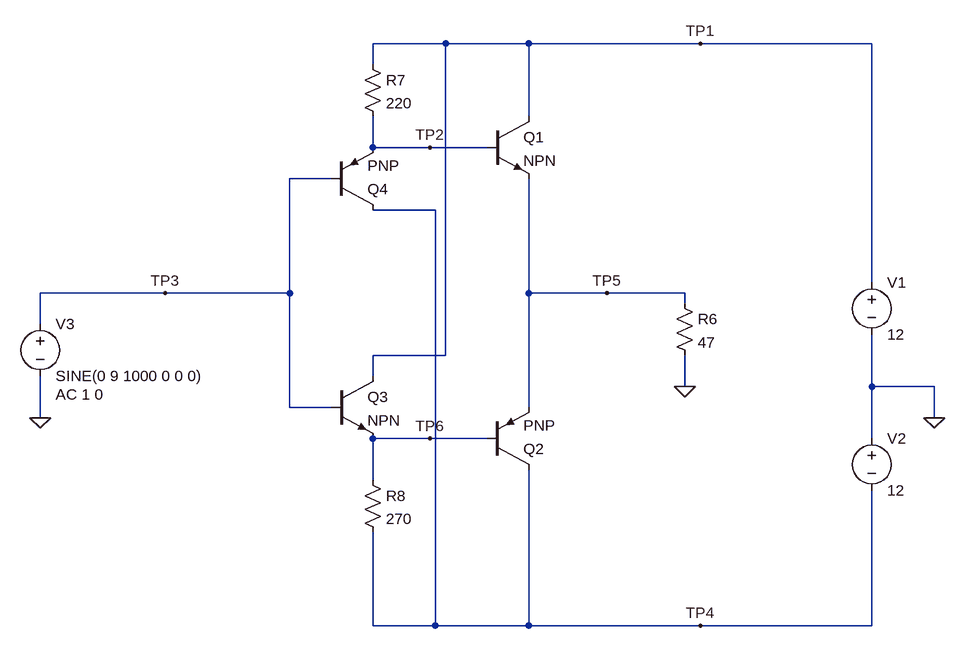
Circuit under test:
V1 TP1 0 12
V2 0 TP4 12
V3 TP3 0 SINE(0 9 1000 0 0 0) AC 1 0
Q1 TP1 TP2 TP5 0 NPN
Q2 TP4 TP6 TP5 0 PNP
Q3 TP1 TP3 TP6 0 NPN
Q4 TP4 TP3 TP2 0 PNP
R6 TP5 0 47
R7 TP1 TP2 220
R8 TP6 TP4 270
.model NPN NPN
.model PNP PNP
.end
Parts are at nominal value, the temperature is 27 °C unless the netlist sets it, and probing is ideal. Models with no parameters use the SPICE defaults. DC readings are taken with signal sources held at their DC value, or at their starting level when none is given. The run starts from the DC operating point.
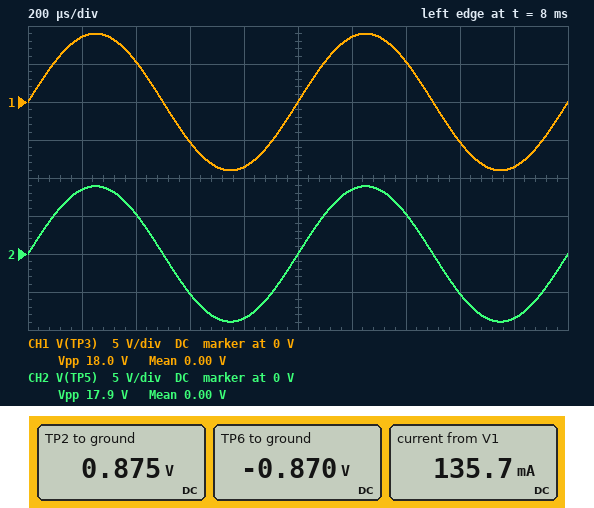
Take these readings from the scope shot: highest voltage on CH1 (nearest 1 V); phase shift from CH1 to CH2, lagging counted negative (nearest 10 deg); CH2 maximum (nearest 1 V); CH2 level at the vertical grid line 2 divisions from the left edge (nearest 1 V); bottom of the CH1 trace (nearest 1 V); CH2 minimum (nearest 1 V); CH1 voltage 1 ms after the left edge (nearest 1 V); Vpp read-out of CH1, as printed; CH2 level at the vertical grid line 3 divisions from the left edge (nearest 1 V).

9 V
0 deg
9 V
5 V
-9 V
-9 V
0 V
18.0 V
-5 V
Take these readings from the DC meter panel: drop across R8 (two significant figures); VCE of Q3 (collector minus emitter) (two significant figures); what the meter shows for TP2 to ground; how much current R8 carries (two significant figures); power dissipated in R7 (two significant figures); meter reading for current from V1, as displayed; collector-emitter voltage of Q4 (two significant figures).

11 V
13 V
0.875 V
41 mA
560 mW
135.7 mA
-13 V
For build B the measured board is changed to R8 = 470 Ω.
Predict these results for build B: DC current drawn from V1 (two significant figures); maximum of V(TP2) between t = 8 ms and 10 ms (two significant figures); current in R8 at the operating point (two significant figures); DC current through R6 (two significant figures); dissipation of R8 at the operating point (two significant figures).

110 mA
9.8 V
24 mA
210 µA
260 mW
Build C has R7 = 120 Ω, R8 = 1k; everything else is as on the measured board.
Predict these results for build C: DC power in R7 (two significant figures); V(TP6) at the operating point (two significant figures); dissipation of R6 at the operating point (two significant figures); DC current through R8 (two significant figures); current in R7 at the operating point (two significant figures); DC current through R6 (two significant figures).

1.0 W
-840 mV
16 µW
11 mA
93 mA
580 µA
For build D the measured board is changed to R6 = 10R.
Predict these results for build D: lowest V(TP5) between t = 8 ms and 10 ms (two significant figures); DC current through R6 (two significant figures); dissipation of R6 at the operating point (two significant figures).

-8.7 V
260 µA
670 nW
